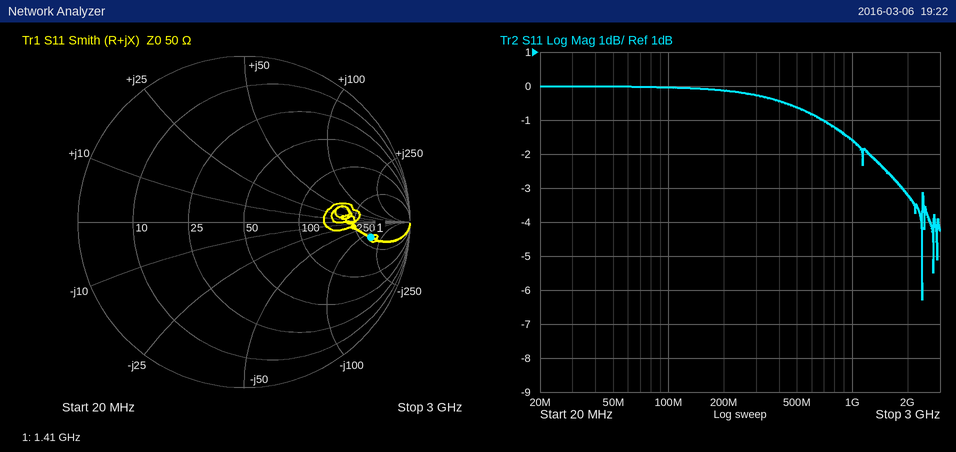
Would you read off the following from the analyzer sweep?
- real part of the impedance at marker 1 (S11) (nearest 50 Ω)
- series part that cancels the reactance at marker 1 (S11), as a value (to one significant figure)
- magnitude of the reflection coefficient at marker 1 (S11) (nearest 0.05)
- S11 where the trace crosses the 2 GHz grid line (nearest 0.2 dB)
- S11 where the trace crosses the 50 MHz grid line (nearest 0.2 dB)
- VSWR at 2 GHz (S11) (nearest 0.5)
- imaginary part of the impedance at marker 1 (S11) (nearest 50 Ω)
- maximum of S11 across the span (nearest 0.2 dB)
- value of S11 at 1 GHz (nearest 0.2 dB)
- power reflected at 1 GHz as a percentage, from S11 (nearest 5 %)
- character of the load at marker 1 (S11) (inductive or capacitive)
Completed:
300 Ω
20 nH
0.75
-3.2 dB
0.0 dB
5.5
-150 Ω
0.0 dB
-1.6 dB
70 %
capacitive
